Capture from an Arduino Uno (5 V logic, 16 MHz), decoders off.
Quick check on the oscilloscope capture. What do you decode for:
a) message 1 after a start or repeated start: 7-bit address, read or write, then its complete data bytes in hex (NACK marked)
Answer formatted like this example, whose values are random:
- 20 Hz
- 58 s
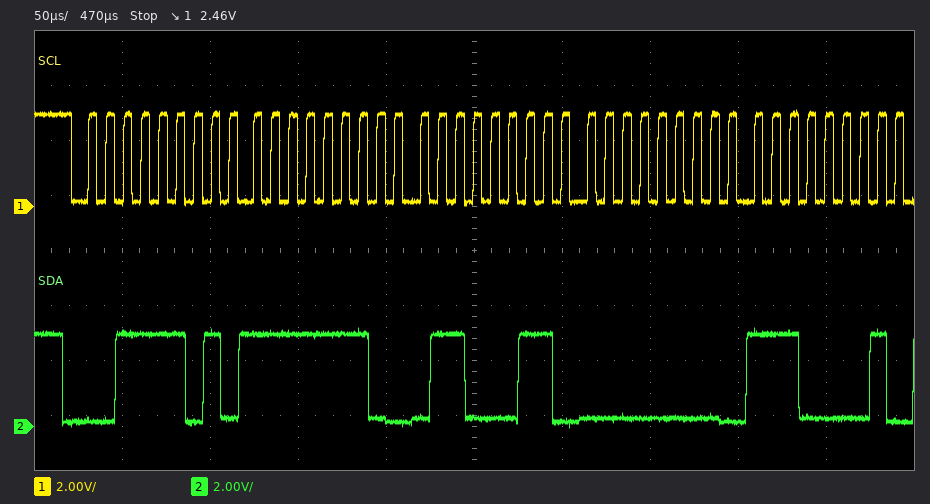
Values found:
- 0x1E read: FE 63 00 E1
